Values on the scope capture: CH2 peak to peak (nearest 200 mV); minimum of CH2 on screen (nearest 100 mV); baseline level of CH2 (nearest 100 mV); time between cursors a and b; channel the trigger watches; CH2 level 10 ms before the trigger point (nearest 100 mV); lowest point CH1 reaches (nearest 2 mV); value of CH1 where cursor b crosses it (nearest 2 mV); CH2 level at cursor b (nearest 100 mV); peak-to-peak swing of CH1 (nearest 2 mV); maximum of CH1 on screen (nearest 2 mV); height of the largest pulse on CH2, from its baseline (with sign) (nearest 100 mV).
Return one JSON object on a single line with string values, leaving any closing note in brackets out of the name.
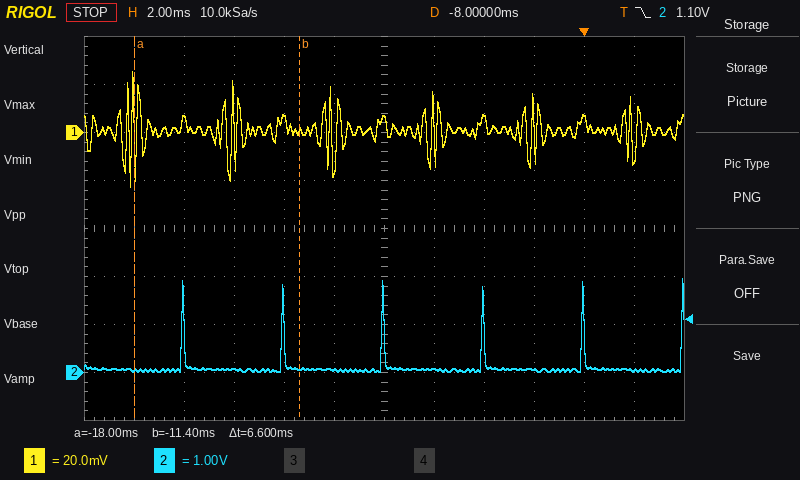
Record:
{"CH2 peak to peak": "2.0 V", "minimum of CH2 on screen": "0.0 V", "baseline level of CH2": "100 mV", "time between cursors a and b": "6.6 ms", "channel the trigger watches": "CH2", "CH2 level 10 ms before the trigger point": "100 mV", "lowest point CH1 reaches": "-22 mV", "value of CH1 where cursor b crosses it": "0 mV", "CH2 level at cursor b": "100 mV", "peak-to-peak swing of CH1": "48 mV", "maximum of CH1 on screen": "26 mV", "height of the largest pulse on CH2, from its baseline (with sign)": "+1.9 V"}
